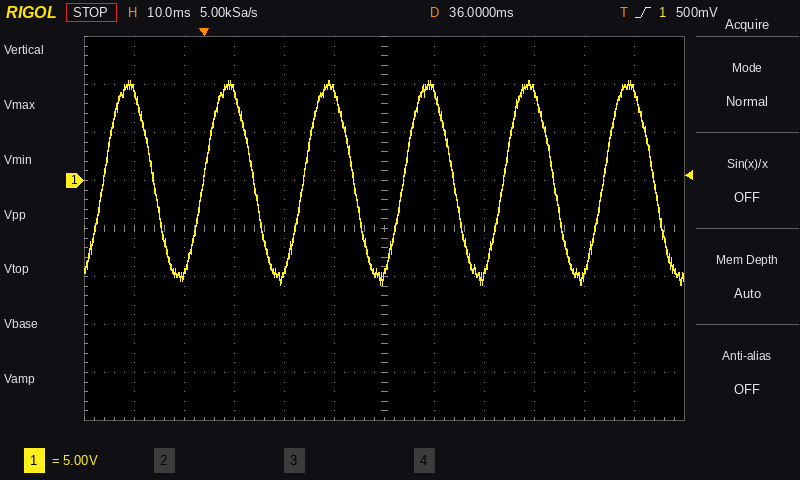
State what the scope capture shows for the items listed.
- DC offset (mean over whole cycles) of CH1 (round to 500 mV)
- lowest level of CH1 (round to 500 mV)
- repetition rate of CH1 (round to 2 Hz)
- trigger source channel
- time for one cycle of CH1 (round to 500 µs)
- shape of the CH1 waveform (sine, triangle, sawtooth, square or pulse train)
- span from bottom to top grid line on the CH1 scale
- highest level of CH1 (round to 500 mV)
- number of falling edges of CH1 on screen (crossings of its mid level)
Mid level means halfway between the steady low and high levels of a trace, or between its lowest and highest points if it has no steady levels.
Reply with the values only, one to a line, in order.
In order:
0.0 V
-11.0 V
50 Hz
CH1
20.0 ms
sine
40 V
10.5 V
6
